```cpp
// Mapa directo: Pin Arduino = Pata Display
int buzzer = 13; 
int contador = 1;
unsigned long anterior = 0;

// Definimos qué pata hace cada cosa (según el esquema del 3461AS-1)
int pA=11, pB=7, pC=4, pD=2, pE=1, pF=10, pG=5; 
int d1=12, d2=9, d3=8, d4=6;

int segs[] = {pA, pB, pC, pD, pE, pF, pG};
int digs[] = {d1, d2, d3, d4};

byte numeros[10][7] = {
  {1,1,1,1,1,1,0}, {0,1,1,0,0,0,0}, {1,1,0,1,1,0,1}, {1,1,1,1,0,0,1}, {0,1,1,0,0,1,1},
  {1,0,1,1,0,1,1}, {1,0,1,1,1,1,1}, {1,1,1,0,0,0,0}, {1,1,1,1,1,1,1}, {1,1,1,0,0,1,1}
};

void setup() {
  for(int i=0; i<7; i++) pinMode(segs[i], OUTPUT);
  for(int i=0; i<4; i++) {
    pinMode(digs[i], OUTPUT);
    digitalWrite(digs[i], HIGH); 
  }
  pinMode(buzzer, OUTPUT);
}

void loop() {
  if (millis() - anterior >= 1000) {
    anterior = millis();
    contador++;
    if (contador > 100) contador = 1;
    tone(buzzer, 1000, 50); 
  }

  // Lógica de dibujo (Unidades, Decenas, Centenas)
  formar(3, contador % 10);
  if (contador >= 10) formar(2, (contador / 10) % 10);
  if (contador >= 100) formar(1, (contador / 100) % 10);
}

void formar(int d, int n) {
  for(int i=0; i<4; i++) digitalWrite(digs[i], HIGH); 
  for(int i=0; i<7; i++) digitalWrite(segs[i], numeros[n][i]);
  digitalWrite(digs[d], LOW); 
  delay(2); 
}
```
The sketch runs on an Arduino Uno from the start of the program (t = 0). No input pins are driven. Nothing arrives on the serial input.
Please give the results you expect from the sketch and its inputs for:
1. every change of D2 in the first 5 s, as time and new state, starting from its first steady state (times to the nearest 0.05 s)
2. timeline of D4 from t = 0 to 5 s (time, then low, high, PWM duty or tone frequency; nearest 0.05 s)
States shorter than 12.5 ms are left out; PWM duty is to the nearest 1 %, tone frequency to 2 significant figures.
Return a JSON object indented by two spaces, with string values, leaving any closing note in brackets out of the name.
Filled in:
{
  "every change of D2 in the first 5 s, as time and new state, starting from its first steady state": "0 s low; 1 s high; 3 s low; 4 s high",
  "timeline of D4 from t = 0 to 5 s": "0 s high; 1 s low; 2 s high"
}
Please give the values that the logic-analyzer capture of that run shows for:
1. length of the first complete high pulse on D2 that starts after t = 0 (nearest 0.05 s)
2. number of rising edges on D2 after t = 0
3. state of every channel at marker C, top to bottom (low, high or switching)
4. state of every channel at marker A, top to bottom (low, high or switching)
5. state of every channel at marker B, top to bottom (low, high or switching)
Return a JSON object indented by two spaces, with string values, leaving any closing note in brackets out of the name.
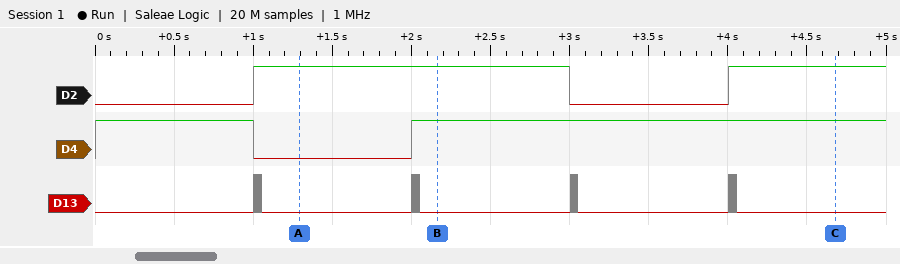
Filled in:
{
  "length of the first complete high pulse on D2 that starts after t = 0": "2.00 s",
  "number of rising edges on D2 after t = 0": "2",
  "state of every channel at marker C, top to bottom": "D2 high, D4 high, D13 low",
  "state of every channel at marker A, top to bottom": "D2 high, D4 low, D13 low",
  "state of every channel at marker B, top to bottom": "D2 high, D4 high, D13 low"
}
